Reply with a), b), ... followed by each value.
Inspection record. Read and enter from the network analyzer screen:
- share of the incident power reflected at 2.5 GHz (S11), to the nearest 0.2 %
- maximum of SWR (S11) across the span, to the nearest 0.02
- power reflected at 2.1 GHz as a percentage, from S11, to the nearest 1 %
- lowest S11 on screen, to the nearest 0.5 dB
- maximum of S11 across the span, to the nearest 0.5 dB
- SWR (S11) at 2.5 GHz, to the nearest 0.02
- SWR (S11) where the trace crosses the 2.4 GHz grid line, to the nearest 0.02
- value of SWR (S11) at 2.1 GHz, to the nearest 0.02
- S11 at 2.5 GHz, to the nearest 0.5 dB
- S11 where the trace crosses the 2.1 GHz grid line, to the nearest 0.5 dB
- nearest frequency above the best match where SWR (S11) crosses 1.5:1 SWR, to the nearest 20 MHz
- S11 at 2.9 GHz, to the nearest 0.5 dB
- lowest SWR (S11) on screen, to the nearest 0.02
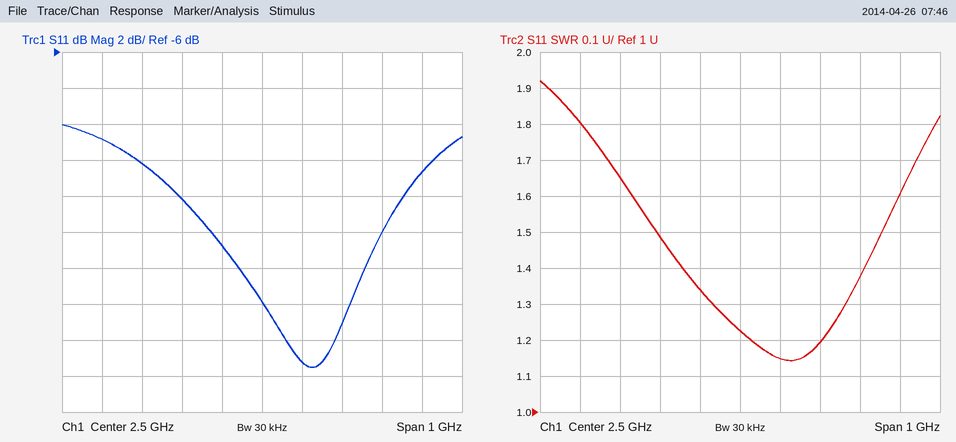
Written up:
a) 1.0 %
b) 1.92
c) 8 %
d) -23.5 dB
e) -10.0 dB
f) 1.22
g) 1.34
h) 1.80
i) -20.0 dB
j) -11.0 dB
k) 2.86 GHz
l) -12.5 dB
m) 1.14
